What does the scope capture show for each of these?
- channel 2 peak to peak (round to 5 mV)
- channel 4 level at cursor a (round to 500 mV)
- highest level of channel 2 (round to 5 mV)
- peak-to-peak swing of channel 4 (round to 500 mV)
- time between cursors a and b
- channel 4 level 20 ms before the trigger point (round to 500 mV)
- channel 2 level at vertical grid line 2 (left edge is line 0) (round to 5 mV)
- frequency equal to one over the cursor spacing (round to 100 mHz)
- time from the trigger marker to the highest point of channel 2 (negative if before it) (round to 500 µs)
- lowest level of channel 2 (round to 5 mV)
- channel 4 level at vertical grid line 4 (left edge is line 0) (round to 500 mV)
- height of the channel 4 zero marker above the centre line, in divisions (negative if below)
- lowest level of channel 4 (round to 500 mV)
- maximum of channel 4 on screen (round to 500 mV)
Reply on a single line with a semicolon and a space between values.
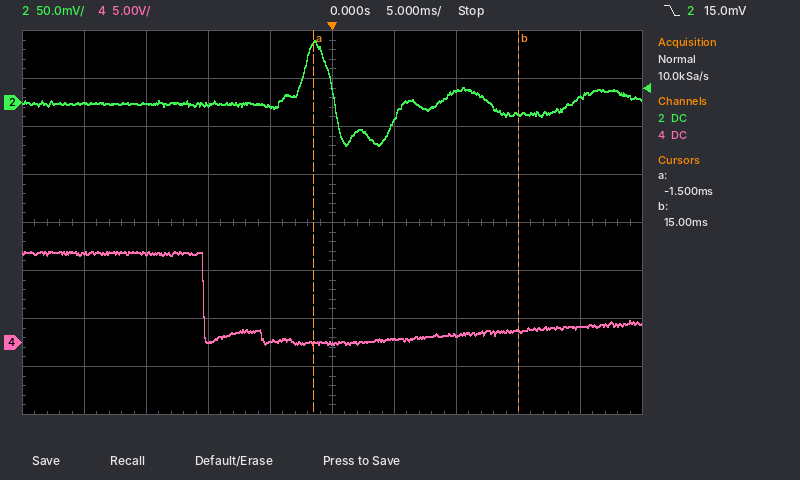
110 mV; 0.0 V; 65 mV; 9.5 V; 16.5 ms; 9.5 V; 0 mV; 60.6 Hz; -1.5 ms; -45 mV; 0.0 V; -2.5 div; 0.0 V; 9.5 V
